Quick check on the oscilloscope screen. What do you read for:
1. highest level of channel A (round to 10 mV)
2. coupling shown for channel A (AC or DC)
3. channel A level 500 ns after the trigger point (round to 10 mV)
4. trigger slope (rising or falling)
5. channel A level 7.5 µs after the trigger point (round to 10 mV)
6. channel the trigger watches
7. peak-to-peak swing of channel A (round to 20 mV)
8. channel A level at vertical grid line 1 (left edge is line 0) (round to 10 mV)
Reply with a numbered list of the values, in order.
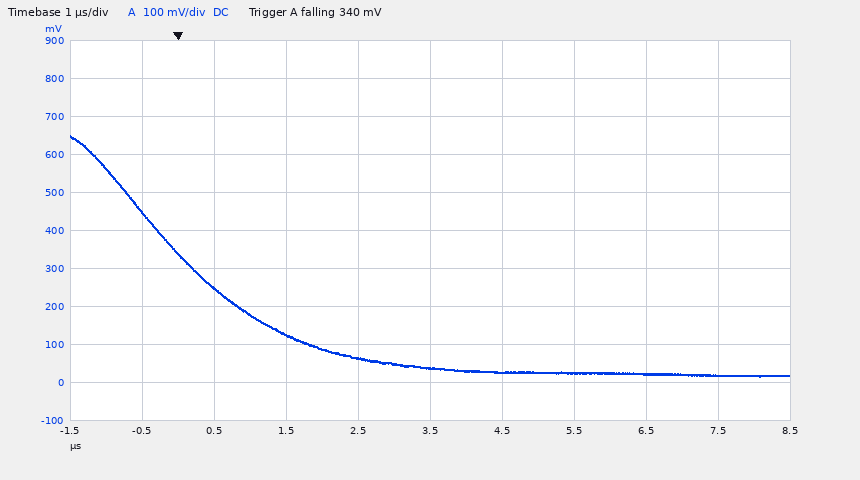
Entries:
1. 650 mV
2. DC
3. 250 mV
4. falling
5. 20 mV
6. channel A
7. 640 mV
8. 450 mV
